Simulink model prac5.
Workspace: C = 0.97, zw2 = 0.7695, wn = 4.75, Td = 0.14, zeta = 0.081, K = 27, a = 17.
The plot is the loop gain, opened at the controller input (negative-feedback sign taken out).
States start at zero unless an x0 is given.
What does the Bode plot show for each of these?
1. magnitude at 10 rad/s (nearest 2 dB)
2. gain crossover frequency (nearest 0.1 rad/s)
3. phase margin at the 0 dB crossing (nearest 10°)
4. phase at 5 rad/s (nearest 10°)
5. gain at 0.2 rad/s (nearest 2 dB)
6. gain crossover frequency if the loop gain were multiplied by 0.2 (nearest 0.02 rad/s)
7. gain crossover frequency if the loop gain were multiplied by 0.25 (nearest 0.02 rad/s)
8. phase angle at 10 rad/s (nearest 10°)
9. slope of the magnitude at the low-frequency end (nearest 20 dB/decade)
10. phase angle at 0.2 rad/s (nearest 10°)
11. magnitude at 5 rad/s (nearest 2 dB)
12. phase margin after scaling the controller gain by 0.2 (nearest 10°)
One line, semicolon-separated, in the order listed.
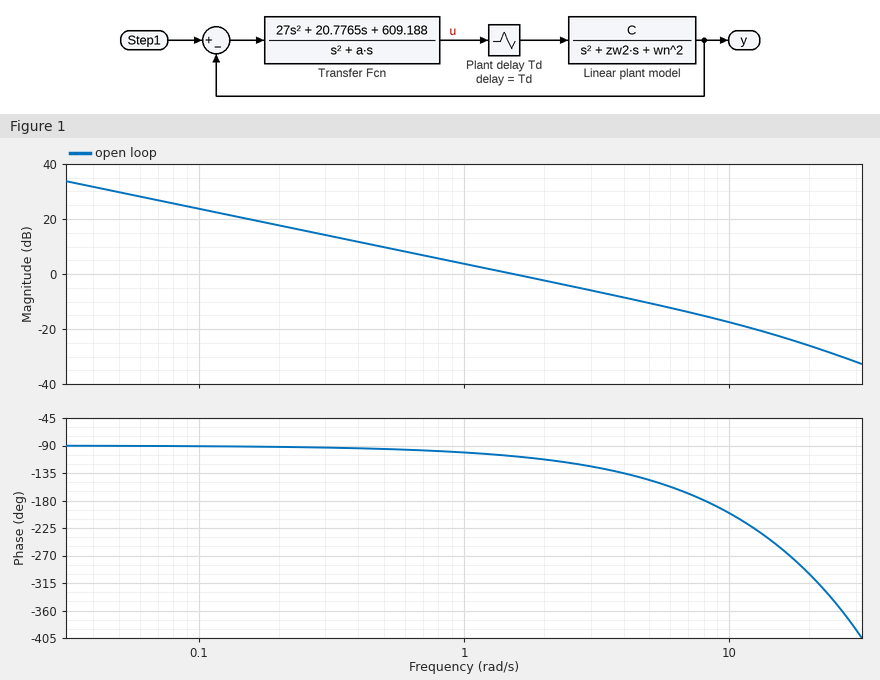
-18 dB; 1.5 rad/s; 70°; -150°; 18 dB; 0.30 rad/s; 0.38 rad/s; -200°; -20 dB/decade; -90°; -10 dB; 90°
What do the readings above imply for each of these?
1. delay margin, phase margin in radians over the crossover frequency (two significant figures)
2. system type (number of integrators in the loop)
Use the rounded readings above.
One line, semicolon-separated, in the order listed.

0.81 s; 1
